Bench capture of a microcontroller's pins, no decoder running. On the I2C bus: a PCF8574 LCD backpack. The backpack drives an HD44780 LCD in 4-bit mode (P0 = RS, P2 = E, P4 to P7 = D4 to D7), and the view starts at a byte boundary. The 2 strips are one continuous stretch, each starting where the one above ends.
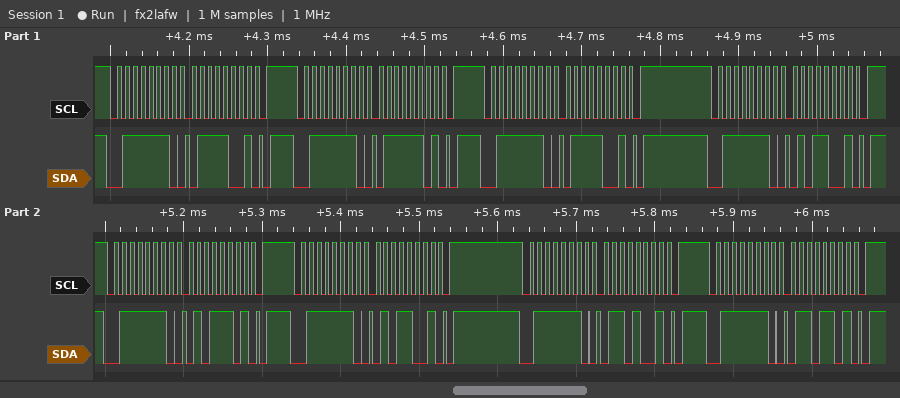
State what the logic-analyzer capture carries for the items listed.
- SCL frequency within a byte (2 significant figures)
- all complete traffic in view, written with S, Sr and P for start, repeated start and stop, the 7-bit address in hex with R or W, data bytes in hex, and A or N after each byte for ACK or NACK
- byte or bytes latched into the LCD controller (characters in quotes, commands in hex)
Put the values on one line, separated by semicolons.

100 kHz; S 3FW A 79 A P S 3FW A 7D A P S 3FW A 79 A P S 3FW A 59 A P S 3FW A 5D A P S 3FW A 59 A P S 3FW A 69 A P S 3FW A 6D A P; 'u'
